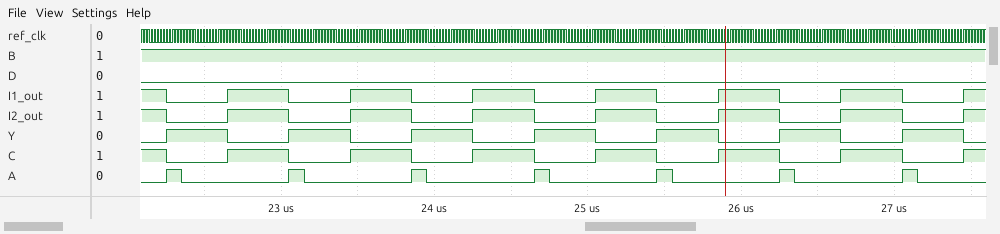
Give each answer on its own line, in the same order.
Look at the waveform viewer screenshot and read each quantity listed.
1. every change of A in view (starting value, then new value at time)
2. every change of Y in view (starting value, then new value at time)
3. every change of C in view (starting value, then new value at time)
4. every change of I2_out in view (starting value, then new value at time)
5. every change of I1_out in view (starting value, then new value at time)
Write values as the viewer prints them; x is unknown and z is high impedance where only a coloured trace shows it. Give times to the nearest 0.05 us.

0, 1 at 22.25 us, 0 at 22.35 us, 1 at 23.05 us, 0 at 23.15 us, 1 at 23.85 us, 0 at 23.95 us, 1 at 24.65 us, 0 at 24.75 us, 1 at 25.45 us, 0 at 25.55 us, 1 at 26.25 us, 0 at 26.35 us, 1 at 27.05 us, 0 at 27.15 us
0, 1 at 22.25 us, 0 at 22.65 us, 1 at 23.05 us, 0 at 23.45 us, 1 at 23.85 us, 0 at 24.25 us, 1 at 24.65 us, 0 at 25.05 us, 1 at 25.45 us, 0 at 25.85 us, 1 at 26.25 us, 0 at 26.65 us, 1 at 27.05 us, 0 at 27.45 us
1, 0 at 22.25 us, 1 at 22.65 us, 0 at 23.05 us, 1 at 23.45 us, 0 at 23.85 us, 1 at 24.25 us, 0 at 24.65 us, 1 at 25.05 us, 0 at 25.45 us, 1 at 25.85 us, 0 at 26.25 us, 1 at 26.65 us, 0 at 27.05 us, 1 at 27.45 us
1, 0 at 22.25 us, 1 at 22.65 us, 0 at 23.05 us, 1 at 23.45 us, 0 at 23.85 us, 1 at 24.25 us, 0 at 24.65 us, 1 at 25.05 us, 0 at 25.45 us, 1 at 25.85 us, 0 at 26.25 us, 1 at 26.65 us, 0 at 27.05 us, 1 at 27.45 us
1, 0 at 22.25 us, 1 at 22.65 us, 0 at 23.05 us, 1 at 23.45 us, 0 at 23.85 us, 1 at 24.25 us, 0 at 24.65 us, 1 at 25.05 us, 0 at 25.45 us, 1 at 25.85 us, 0 at 26.25 us, 1 at 26.65 us, 0 at 27.05 us, 1 at 27.45 us
